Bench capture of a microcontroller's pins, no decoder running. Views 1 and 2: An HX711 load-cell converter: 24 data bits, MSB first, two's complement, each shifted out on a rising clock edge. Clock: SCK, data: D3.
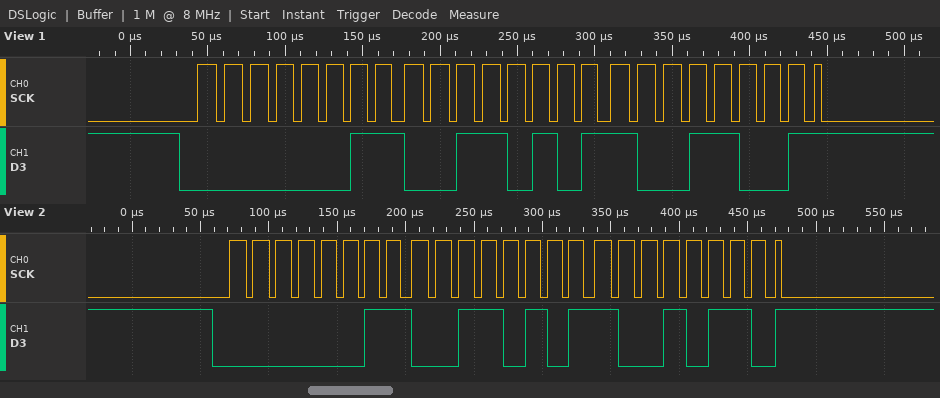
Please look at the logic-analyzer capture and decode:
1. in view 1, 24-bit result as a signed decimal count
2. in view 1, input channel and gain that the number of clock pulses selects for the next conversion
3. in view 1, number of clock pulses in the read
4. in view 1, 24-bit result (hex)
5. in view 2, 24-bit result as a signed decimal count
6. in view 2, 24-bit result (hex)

210329
channel A, gain 128
25
0x033599
210326
0x033596
